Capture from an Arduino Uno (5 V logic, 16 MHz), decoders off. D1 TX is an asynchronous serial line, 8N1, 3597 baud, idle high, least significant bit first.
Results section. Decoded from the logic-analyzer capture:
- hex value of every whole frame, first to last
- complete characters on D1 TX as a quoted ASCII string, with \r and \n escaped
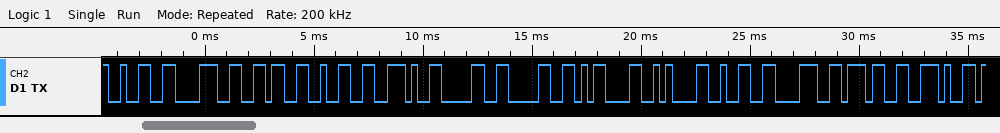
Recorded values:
32 38 36 32 2E 30 30 0D 0A 32 38 37 2E
"2862.00\r\n287."
